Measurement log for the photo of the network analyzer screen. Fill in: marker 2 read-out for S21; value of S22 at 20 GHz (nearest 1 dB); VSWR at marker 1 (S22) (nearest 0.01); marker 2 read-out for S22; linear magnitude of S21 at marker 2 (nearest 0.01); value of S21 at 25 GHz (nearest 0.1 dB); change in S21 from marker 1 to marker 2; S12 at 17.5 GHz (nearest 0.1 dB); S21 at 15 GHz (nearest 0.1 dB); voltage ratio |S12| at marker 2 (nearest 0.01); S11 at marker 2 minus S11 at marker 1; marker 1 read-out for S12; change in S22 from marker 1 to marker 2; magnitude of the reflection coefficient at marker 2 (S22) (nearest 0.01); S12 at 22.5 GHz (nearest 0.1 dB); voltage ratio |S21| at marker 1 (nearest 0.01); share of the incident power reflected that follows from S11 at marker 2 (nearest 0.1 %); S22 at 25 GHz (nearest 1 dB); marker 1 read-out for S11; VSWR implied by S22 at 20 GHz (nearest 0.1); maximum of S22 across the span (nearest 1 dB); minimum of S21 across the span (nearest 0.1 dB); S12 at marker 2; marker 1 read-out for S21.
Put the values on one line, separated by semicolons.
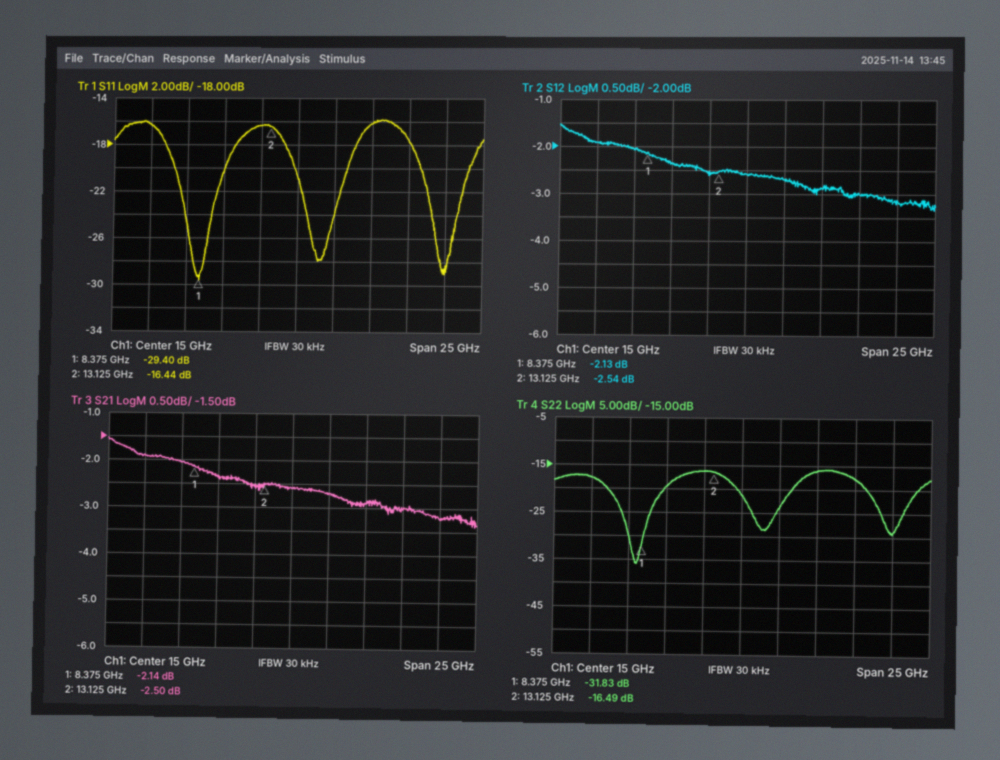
-2.50 dB; -16 dB; 1.05; -16.49 dB; 0.75; -3.2 dB; -0.36 dB; -2.7 dB; -2.6 dB; 0.75; 12.96 dB; -2.13 dB; 15.34 dB; 0.15; -3.0 dB; 0.78; 2.3 %; -29 dB; -29.40 dB; 1.4; -16 dB; -3.4 dB; -2.54 dB; -2.14 dB
